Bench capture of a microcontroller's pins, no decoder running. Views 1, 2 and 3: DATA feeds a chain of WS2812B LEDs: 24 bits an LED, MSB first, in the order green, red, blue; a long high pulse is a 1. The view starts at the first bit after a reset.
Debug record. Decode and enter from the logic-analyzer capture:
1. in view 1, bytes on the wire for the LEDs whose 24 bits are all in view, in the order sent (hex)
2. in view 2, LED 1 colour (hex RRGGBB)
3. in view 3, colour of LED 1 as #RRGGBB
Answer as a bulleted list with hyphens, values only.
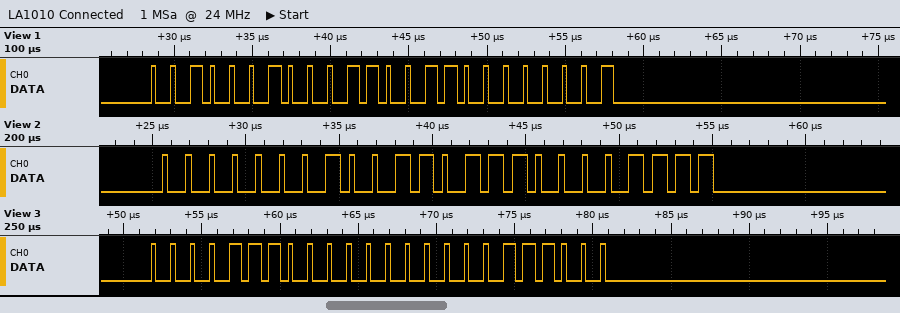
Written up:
- 22 33 01
- #37010F
- #000E38
